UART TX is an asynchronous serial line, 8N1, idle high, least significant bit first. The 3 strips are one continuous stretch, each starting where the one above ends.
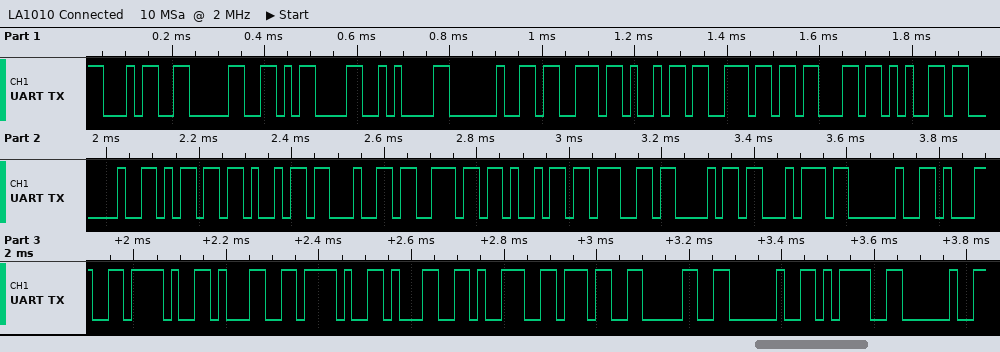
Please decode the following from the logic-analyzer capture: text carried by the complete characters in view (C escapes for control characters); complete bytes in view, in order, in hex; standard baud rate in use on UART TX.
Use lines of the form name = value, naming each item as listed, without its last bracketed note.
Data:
text carried by the complete characters in view = "40\r\n since midnight 1/1/1970 = "
complete bytes in view, in order, in hex = 34 30 0D 0A 20 73 69 6E 63 65 20 6D 69 64 6E 69 67 68 74 20 31 2F 31 2F 31 39 37 30 20 3D 20
standard baud rate in use on UART TX = 57600 baud
